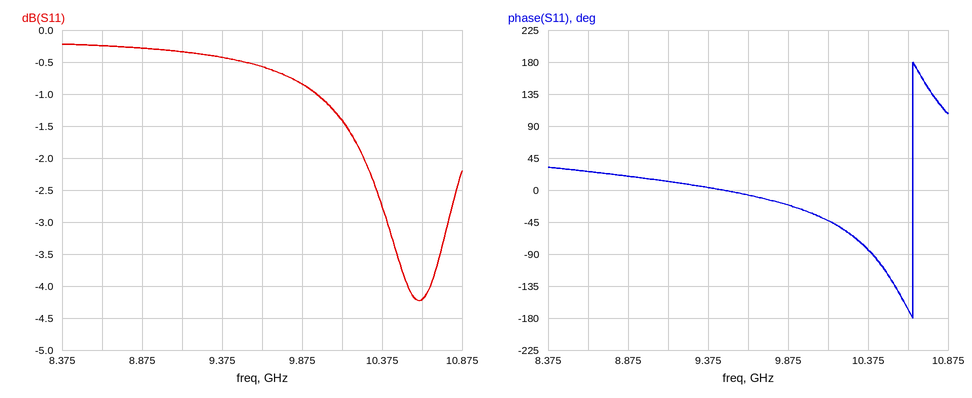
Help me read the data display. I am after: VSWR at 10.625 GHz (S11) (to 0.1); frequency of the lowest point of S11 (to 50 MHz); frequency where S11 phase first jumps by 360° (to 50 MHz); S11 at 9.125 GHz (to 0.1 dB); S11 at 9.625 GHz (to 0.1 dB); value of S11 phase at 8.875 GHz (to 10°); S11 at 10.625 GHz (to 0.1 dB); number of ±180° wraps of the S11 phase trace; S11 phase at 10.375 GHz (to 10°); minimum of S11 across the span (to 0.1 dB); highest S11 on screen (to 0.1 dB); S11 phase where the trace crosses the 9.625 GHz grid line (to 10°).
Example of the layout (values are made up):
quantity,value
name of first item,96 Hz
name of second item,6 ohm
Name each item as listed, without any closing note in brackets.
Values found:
quantity,value
VSWR at 10.625 GHz (S11),4.2
frequency of the lowest point of S11,10.60 GHz
frequency where S11 phase first jumps by 360°,10.65 GHz
S11 at 9.125 GHz,-0.3 dB
S11 at 9.625 GHz,-0.6 dB
value of S11 phase at 8.875 GHz,20°
S11 at 10.625 GHz,-4.2 dB
number of ±180° wraps of the S11 phase trace,1
S11 phase at 10.375 GHz,-80°
minimum of S11 across the span,-4.2 dB
highest S11 on screen,-0.2 dB
S11 phase where the trace crosses the 9.625 GHz grid line,-10°
